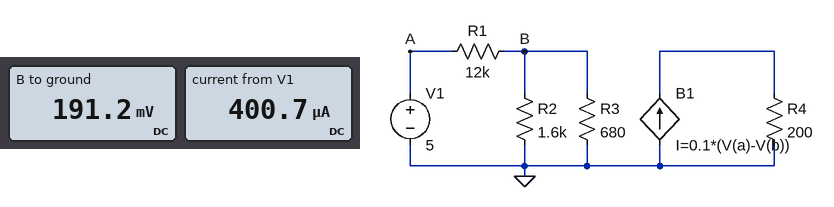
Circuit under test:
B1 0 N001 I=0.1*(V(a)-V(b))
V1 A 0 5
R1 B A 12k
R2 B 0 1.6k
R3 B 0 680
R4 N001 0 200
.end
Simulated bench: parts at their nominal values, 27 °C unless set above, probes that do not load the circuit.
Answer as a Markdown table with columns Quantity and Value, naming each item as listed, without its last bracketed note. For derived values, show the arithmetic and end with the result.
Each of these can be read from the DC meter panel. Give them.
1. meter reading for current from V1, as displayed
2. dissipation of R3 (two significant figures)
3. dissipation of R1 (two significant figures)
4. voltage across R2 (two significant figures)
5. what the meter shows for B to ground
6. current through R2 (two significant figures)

| Quantity | Value |
|---|---|
| meter reading for current from V1, as displayed | 400.7 µA |
| dissipation of R3 | (191.2 mV)^2 / 680 Ω = 54 µW |
| dissipation of R1 | (5 V - 191.2 mV)^2 / 12 kΩ = 1.9 mW |
| voltage across R2 | 191.2 mV = 190 mV |
| what the meter shows for B to ground | 191.2 mV |
| current through R2 | (191.2 mV) / 1.6 kΩ = 120 µA |
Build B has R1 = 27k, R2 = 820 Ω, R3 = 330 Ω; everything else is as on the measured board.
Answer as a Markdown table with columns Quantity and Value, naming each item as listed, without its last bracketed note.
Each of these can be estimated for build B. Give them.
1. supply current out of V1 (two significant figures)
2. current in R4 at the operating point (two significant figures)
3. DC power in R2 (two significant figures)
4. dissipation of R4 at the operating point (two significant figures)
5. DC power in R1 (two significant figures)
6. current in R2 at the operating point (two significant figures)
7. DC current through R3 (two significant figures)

| Quantity | Value |
|---|---|
| supply current out of V1 | 180 µA |
| current in R4 at the operating point | 500 mA |
| DC power in R2 | 2.3 µW |
| dissipation of R4 at the operating point | 49 W |
| DC power in R1 | 910 µW |
| current in R2 at the operating point | 53 µA |
| DC current through R3 | 130 µA |
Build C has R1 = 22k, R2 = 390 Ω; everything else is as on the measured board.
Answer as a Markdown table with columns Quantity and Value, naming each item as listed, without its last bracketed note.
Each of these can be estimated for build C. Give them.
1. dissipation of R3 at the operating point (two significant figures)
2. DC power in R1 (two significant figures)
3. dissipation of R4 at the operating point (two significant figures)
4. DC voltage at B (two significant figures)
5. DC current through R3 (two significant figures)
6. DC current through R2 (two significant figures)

| Quantity | Value |
|---|---|
| dissipation of R3 at the operating point | 4.6 µW |
| DC power in R1 | 1.1 mW |
| dissipation of R4 at the operating point | 49 W |
| DC voltage at B | 56 mV |
| DC current through R3 | 82 µA |
| DC current through R2 | 140 µA |
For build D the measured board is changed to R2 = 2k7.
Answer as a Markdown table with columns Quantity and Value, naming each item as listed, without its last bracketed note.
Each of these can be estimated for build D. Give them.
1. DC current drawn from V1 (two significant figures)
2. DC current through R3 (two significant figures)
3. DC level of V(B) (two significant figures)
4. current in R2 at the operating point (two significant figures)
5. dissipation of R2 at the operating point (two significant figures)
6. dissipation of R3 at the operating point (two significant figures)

| Quantity | Value |
|---|---|
| DC current drawn from V1 | 400 µA |
| DC current through R3 | 320 µA |
| DC level of V(B) | 220 mV |
| current in R2 at the operating point | 80 µA |
| dissipation of R2 at the operating point | 17 µW |
| dissipation of R3 at the operating point | 69 µW |
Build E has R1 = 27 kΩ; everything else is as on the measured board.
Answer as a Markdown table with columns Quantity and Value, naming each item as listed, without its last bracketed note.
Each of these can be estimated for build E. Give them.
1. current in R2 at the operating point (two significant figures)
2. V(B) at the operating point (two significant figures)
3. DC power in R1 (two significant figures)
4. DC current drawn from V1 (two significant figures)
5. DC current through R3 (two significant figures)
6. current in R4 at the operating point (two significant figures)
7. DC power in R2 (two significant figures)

| Quantity | Value |
|---|---|
| current in R2 at the operating point | 54 µA |
| V(B) at the operating point | 87 mV |
| DC power in R1 | 890 µW |
| DC current drawn from V1 | 180 µA |
| DC current through R3 | 130 µA |
| current in R4 at the operating point | 490 mA |
| DC power in R2 | 4.7 µW |
